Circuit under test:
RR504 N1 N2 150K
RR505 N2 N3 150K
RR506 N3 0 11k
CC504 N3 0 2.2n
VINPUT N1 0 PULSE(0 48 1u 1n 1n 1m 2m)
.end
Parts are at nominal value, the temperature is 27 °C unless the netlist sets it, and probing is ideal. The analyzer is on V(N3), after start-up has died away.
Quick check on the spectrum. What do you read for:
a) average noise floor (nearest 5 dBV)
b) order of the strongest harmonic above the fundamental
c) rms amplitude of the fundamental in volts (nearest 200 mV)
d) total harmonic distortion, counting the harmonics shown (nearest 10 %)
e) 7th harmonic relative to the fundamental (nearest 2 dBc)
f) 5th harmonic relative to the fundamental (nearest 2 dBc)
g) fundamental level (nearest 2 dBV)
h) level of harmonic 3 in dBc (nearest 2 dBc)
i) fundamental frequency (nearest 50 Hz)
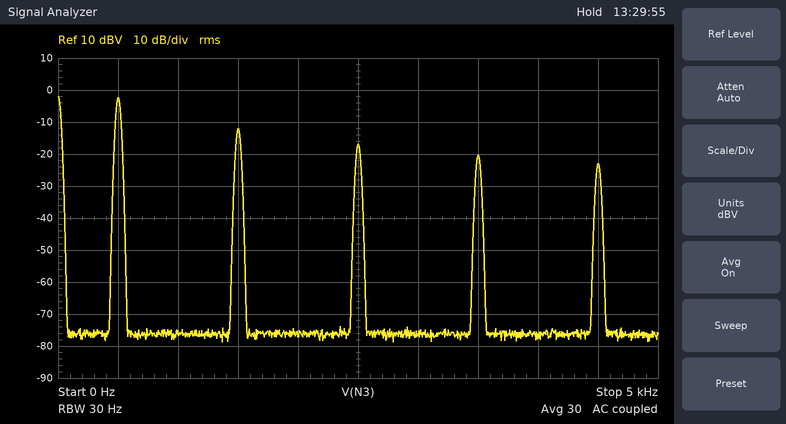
-75 dBV
3
800 mV
40 %
-18 dBc
-14 dBc
-2 dBV
-10 dBc
500 Hz
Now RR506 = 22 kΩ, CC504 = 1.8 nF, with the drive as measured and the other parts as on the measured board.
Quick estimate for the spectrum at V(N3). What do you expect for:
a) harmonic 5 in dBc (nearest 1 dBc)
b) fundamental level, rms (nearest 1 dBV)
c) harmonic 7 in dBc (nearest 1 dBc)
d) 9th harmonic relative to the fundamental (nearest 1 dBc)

-15 dBc
3 dBV
-19 dBc
-22 dBc
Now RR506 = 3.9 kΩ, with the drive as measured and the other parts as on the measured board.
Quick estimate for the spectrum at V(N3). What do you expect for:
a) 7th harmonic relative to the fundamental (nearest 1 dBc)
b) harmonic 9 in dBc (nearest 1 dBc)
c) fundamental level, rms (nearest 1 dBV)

-17 dBc
-19 dBc
-11 dBV
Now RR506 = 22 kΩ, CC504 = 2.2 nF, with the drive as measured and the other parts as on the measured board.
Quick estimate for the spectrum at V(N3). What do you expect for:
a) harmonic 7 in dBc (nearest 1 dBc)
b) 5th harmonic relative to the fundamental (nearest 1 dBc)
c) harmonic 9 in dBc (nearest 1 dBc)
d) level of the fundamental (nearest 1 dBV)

-20 dBc
-16 dBc
-23 dBc
3 dBV
